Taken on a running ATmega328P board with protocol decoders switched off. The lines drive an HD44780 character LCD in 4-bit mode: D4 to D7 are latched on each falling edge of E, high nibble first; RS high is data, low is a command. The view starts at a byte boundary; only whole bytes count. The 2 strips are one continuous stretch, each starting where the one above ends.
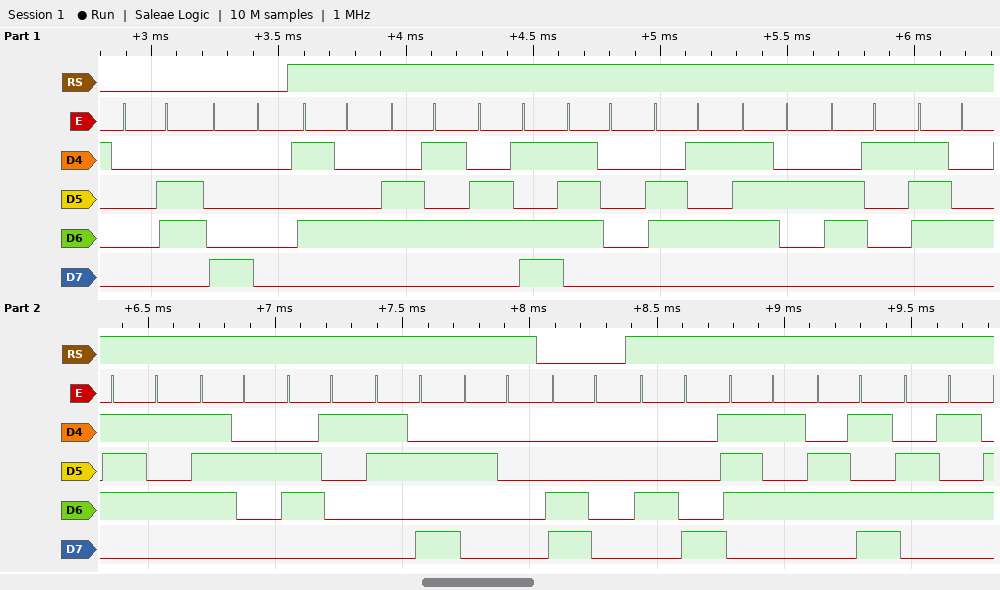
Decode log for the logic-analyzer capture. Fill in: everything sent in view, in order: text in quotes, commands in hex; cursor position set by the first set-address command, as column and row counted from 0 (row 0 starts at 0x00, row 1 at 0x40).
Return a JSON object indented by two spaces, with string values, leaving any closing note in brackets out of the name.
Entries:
{
  "everything sent in view, in order: text in quotes, commands in hex": "0x06 0x80 \"Temperatura: \" 0xC0 \"Hume\"",
  "cursor position set by the first set-address command, as column and row counted from 0": "column 0, row 0"
}
